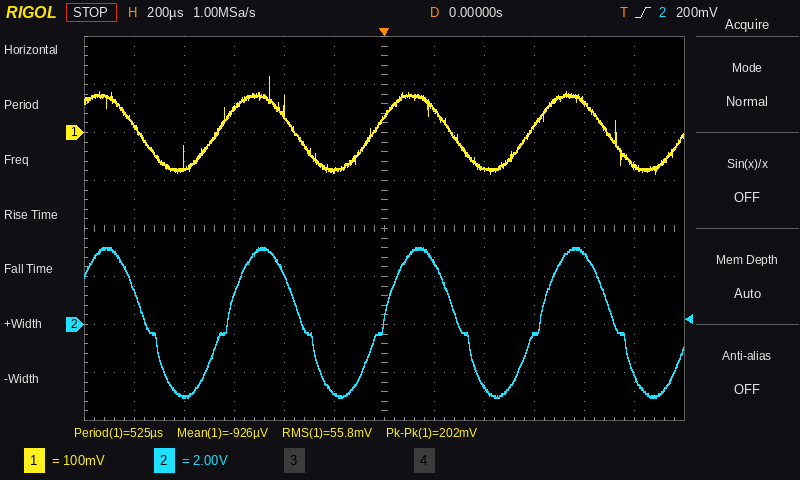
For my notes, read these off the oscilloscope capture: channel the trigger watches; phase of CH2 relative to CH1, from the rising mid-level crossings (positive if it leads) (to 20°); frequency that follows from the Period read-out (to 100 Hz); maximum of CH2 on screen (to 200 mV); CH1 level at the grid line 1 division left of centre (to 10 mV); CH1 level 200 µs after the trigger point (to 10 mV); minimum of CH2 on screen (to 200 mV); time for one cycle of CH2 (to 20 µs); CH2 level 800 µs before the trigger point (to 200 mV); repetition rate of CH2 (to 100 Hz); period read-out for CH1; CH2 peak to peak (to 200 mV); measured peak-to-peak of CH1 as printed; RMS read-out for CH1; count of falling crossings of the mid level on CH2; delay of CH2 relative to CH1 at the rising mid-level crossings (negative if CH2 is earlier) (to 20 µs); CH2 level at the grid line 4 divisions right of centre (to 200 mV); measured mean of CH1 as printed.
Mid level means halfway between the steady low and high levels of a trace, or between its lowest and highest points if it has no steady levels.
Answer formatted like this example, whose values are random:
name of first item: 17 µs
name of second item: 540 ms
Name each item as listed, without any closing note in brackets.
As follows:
channel the trigger watches: CH2
phase of CH2 relative to CH1, from the rising mid-level crossings (positive if it leads): -20°
frequency that follows from the Period read-out: 1.9 kHz
maximum of CH2 on screen: 3.2 V
CH1 level at the grid line 1 division left of centre: -80 mV
CH1 level 200 µs after the trigger point: 50 mV
minimum of CH2 on screen: -3.0 V
time for one cycle of CH2: 620 µs
CH2 level 800 µs before the trigger point: -3.0 V
repetition rate of CH2: 1.6 kHz
period read-out for CH1: 525 µs
CH2 peak to peak: 6.2 V
measured peak-to-peak of CH1 as printed: 202 mV
RMS read-out for CH1: 55.8 mV
count of falling crossings of the mid level on CH2: 4
delay of CH2 relative to CH1 at the rising mid-level crossings (negative if CH2 is earlier): +20 µs
CH2 level at the grid line 4 divisions right of centre: 3.0 V
measured mean of CH1 as printed: -926 µV
